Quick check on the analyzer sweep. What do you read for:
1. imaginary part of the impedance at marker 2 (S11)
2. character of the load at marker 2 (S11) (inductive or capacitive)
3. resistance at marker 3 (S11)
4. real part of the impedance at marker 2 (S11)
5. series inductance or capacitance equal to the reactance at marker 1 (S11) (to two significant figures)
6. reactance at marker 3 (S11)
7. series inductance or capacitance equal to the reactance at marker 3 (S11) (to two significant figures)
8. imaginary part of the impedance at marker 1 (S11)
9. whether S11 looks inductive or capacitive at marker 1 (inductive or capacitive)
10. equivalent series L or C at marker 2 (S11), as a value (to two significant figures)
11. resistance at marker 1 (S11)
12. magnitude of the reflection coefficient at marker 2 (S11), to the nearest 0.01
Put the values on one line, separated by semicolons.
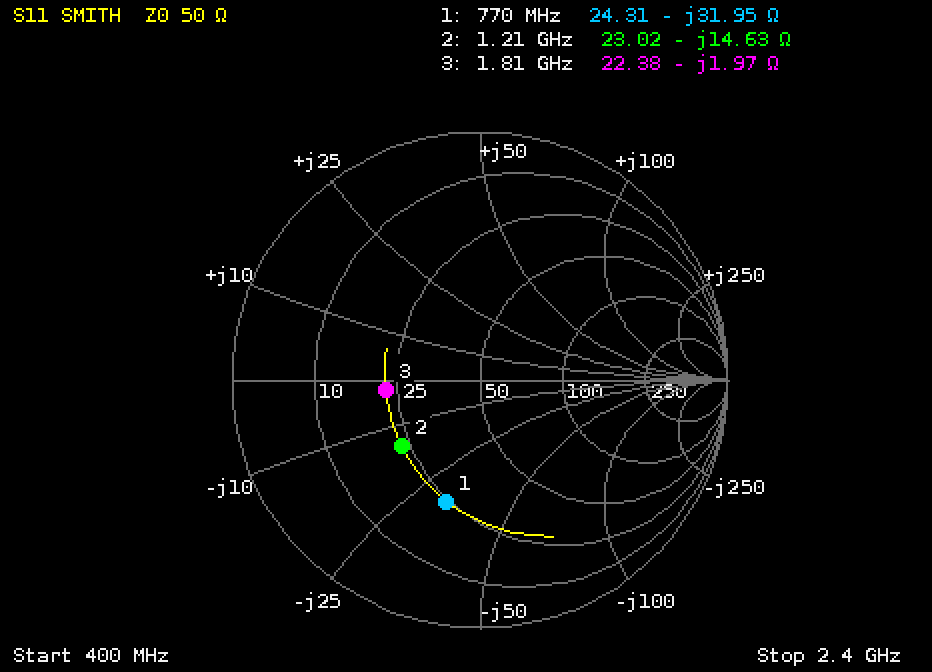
-14.63 Ω; capacitive; 22.38 Ω; 23.02 Ω; 6.5 pF; -1.97 Ω; 45 pF; -31.95 Ω; capacitive; 9.0 pF; 24.31 Ω; 0.41
